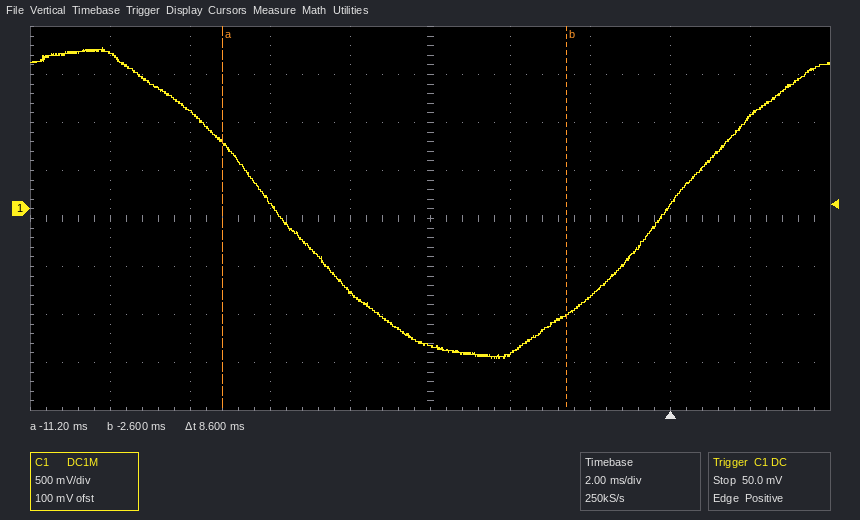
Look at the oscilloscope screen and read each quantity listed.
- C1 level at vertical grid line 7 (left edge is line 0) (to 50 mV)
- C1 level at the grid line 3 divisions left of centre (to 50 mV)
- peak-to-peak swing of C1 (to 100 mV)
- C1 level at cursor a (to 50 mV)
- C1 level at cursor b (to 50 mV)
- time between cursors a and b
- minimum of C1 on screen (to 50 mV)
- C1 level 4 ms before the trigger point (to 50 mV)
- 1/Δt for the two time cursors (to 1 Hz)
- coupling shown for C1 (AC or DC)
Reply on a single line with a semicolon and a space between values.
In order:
-900 mV; 1.00 V; 3.20 V; 700 mV; -1.10 V; 8.6 ms; -1.55 V; -1.50 V; 116 Hz; DC
